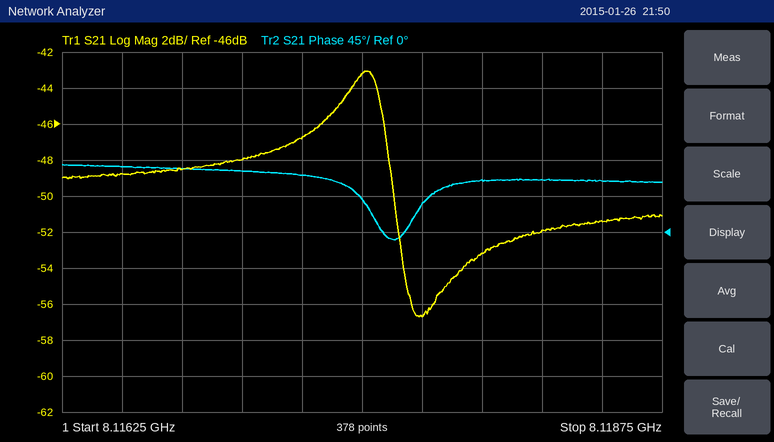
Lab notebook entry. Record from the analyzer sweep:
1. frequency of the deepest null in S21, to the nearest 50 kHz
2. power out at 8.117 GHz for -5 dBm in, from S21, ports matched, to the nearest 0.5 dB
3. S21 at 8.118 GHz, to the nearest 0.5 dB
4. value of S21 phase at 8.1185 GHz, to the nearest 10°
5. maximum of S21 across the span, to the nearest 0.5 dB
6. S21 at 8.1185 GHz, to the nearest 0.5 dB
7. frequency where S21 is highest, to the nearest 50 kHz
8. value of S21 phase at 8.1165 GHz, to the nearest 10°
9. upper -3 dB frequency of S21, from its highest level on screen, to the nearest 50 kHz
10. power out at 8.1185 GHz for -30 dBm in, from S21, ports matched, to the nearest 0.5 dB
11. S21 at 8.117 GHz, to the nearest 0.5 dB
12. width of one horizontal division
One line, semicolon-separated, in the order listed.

8.11775 GHz; -53.0 dBm; -53.0 dB; 60°; -43.0 dB; -51.5 dB; 8.11750 GHz; 80°; 8.11760 GHz; -81.5 dBm; -48.0 dB; 250 kHz
